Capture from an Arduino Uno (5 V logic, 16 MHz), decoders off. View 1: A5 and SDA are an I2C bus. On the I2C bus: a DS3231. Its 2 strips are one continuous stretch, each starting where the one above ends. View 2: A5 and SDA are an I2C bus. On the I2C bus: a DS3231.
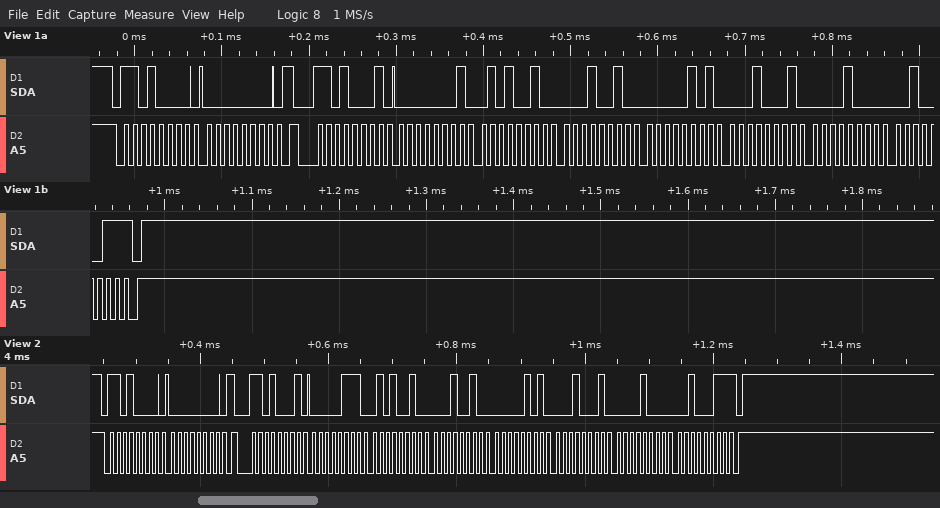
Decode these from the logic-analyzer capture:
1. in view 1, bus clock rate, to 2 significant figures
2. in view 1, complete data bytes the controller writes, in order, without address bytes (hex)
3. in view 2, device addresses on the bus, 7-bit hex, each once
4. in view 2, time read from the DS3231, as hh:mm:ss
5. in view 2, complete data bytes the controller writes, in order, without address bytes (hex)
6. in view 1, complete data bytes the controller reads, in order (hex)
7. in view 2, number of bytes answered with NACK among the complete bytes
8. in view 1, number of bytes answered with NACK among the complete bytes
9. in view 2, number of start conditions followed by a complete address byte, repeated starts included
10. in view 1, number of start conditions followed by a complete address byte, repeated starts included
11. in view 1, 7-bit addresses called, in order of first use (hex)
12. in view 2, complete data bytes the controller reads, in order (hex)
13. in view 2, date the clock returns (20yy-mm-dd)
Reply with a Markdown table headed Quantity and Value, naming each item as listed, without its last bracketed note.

| Quantity | Value |
|---|---|
| in view 1, bus clock rate, to 2 significant figures | 100 kHz |
| in view 1, complete data bytes the controller writes, in order, without address bytes | 00 |
| in view 2, device addresses on the bus, 7-bit hex, each once | 0x68 |
| in view 2, time read from the DS3231, as hh:mm:ss | 12:52:07 |
| in view 2, complete data bytes the controller writes, in order, without address bytes | 00 |
| in view 1, complete data bytes the controller reads, in order | 01 52 12 05 11 08 23 |
| in view 2, number of bytes answered with NACK among the complete bytes | 1 |
| in view 1, number of bytes answered with NACK among the complete bytes | 1 |
| in view 2, number of start conditions followed by a complete address byte, repeated starts included | 2 |
| in view 1, number of start conditions followed by a complete address byte, repeated starts included | 2 |
| in view 1, 7-bit addresses called, in order of first use | 0x68 |
| in view 2, complete data bytes the controller reads, in order | 07 52 12 05 11 08 23 |
| in view 2, date the clock returns | 2023-08-11 |
